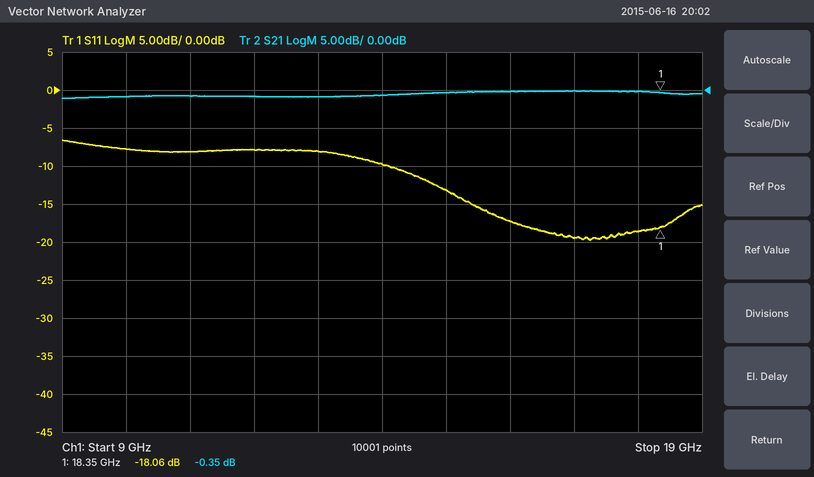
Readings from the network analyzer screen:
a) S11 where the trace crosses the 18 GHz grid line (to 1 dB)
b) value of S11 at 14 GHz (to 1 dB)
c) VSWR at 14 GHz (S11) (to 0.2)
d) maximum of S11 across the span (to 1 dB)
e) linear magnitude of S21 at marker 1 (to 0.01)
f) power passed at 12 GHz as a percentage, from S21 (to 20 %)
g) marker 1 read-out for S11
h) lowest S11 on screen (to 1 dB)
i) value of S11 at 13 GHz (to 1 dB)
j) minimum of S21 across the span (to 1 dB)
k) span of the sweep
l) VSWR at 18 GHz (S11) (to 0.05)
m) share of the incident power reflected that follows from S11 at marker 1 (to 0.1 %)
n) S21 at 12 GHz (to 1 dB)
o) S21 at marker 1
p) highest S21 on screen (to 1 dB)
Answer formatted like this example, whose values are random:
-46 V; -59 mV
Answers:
-19 dB; -10 dB; 2.0; -7 dB; 0.96; 80 %; -18.06 dB; -20 dB; -8 dB; -1 dB; 10 GHz; 1.25; 1.6 %; -1 dB; -0.35 dB; 0 dB
